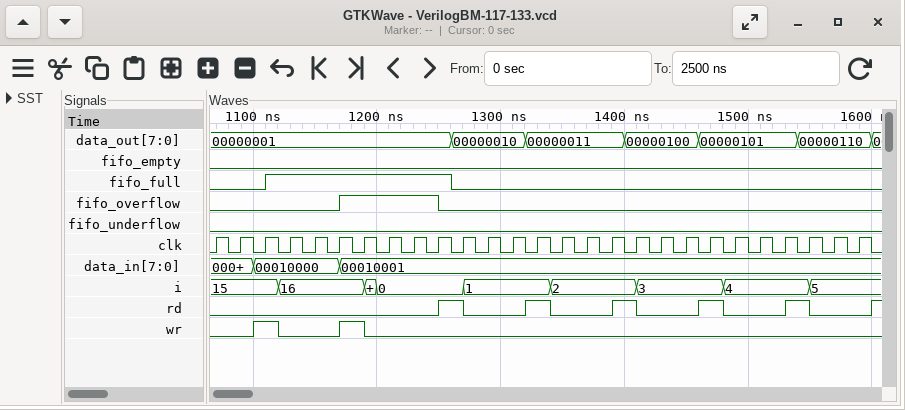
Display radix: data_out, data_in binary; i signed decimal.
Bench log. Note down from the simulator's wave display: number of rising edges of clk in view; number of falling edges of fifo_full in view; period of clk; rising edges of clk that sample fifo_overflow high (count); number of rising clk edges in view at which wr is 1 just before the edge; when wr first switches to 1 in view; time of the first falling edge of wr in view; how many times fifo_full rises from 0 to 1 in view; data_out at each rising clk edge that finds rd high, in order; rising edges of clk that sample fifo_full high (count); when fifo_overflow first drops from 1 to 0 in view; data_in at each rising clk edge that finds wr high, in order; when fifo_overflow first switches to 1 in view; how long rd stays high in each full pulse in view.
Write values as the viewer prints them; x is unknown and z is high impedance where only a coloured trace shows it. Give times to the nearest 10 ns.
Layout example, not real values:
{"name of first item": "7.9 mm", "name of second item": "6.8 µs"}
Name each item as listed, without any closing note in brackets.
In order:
{"number of rising edges of clk in view": "27", "number of falling edges of fifo_full in view": "1", "period of clk": "20 ns", "rising edges of clk that sample fifo_overflow high": "4", "number of rising clk edges in view at which wr is 1 just before the edge": "2", "when wr first switches to 1 in view": "1100 ns", "time of the first falling edge of wr in view": "1120 ns", "how many times fifo_full rises from 0 to 1 in view": "1", "data_out at each rising clk edge that finds rd high, in order": "00000010, 00000011, 00000100, 00000101, 00000110", "rising edges of clk that sample fifo_full high": "7", "when fifo_overflow first drops from 1 to 0 in view": "1250 ns", "data_in at each rising clk edge that finds wr high, in order": "00010000, 00010001", "when fifo_overflow first switches to 1 in view": "1170 ns", "how long rd stays high in each full pulse in view": "20 ns, 20 ns, 20 ns, 20 ns, 20 ns"}
